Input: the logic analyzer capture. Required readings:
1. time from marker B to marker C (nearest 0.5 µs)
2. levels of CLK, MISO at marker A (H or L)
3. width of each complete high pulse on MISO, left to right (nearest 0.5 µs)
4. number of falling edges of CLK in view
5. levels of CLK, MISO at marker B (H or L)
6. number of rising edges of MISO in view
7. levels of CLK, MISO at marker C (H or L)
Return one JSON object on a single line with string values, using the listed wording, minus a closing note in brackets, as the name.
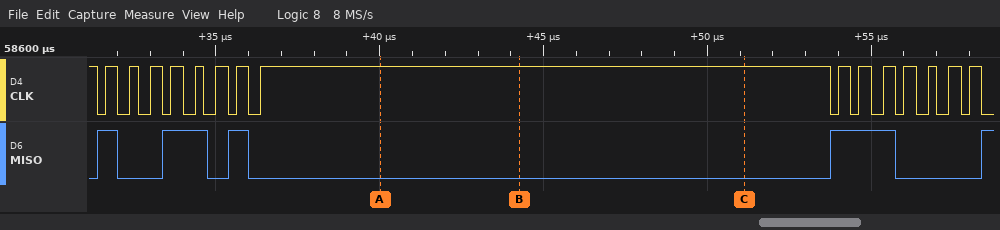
{"time from marker B to marker C": "7 µs", "levels of CLK, MISO at marker A": "CLK=H, MISO=L", "width of each complete high pulse on MISO, left to right": "0.5 µs, 1.5 µs, 0.5 µs, 2 µs", "number of falling edges of CLK in view": "16", "levels of CLK, MISO at marker B": "CLK=H, MISO=L", "number of rising edges of MISO in view": "5", "levels of CLK, MISO at marker C": "CLK=H, MISO=L"}
